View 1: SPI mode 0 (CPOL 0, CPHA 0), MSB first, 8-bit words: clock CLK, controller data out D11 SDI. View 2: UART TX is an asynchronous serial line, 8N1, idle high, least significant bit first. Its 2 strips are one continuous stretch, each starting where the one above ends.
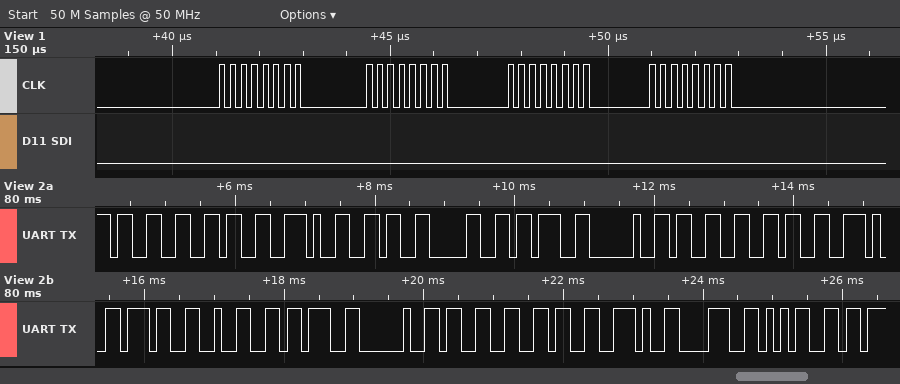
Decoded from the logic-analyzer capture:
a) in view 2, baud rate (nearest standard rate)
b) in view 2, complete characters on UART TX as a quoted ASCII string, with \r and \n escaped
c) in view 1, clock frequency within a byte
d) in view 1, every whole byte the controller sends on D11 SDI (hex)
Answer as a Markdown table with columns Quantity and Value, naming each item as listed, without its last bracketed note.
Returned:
| Quantity | Value |
|---|---|
| in view 2, baud rate | 9600 baud |
| in view 2, complete characters on UART TX as a quoted ASCII string, with \r and \n escaped | "36.60; 36.72; 36.85" |
| in view 1, clock frequency within a byte | 4 MHz |
| in view 1, every whole byte the controller sends on D11 SDI | 0x00 0x00 0x00 0x00 |
